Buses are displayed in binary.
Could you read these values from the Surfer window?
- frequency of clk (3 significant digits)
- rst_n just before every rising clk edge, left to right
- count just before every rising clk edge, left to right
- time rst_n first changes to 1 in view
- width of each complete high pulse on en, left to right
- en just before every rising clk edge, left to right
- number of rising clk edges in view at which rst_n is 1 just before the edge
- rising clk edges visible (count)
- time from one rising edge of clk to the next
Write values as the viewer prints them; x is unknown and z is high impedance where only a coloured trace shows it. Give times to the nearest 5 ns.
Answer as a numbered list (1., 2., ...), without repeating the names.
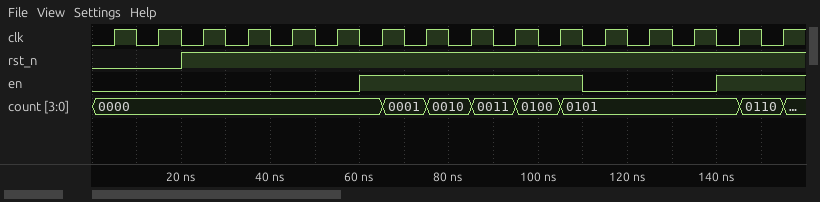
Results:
1. 100 MHz
2. 0 0 1 1 1 1 1 1 1 1 1 1 1 1 1 1
3. 0000, 0000, 0000, 0000, 0000, 0000, 0000, 0001, 0010, 0011, 0100, 0101, 0101, 0101, 0101, 0110
4. 20 ns
5. 50 ns
6. 0 0 0 0 0 0 1 1 1 1 1 0 0 0 1 1
7. 14
8. 16
9. 10 ns
